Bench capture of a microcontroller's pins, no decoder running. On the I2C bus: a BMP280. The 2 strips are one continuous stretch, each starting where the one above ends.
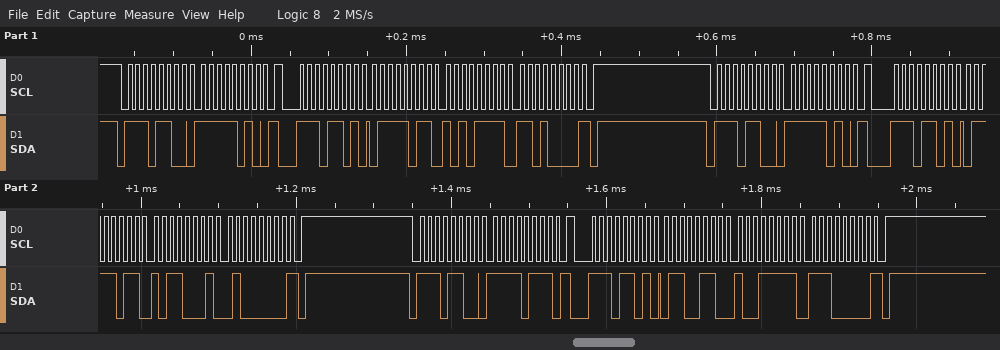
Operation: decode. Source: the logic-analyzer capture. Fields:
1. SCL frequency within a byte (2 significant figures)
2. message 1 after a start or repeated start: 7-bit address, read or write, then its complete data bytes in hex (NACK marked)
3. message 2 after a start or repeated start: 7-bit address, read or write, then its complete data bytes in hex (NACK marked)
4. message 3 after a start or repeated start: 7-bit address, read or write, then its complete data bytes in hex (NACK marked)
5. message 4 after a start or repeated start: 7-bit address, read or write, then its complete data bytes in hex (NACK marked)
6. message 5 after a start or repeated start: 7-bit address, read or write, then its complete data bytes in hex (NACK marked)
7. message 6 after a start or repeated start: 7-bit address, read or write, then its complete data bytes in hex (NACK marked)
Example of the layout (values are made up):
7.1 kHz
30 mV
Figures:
100 kHz
0x76 write: FA
0x76 read: 7B AF D0 NACK
0x76 write: FA
0x76 read: 7B B1 40 NACK
0x76 write: F7
0x76 read: 66 9F E0 NACK
